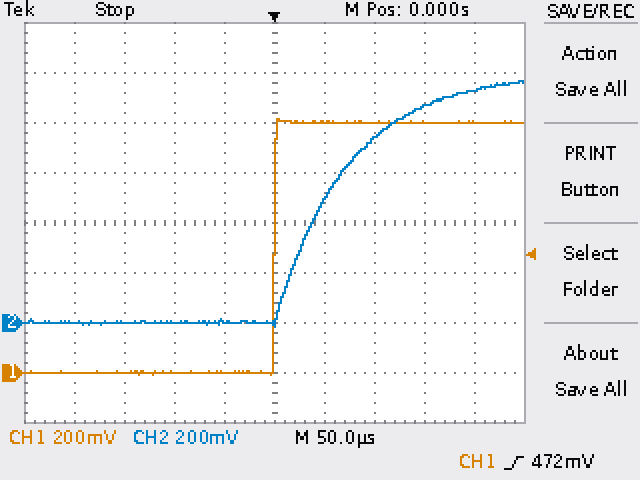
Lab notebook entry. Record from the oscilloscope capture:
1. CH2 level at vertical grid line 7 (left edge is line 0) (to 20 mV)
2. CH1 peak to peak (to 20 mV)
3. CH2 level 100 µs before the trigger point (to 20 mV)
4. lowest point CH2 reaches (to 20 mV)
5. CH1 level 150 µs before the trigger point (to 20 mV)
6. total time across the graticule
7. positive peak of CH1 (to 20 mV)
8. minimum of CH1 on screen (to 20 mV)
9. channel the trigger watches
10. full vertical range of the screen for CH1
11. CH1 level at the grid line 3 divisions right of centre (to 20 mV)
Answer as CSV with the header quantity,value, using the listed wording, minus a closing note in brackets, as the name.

quantity,value
CH2 level at vertical grid line 7 (left edge is line 0),740 mV
CH1 peak to peak,1.02 V
CH2 level 100 µs before the trigger point,0 mV
lowest point CH2 reaches,-20 mV
CH1 level 150 µs before the trigger point,0 mV
total time across the graticule,500 µs
positive peak of CH1,1.02 V
minimum of CH1 on screen,0 mV
channel the trigger watches,CH1
full vertical range of the screen for CH1,1.6 V
CH1 level at the grid line 3 divisions right of centre,1.00 V
